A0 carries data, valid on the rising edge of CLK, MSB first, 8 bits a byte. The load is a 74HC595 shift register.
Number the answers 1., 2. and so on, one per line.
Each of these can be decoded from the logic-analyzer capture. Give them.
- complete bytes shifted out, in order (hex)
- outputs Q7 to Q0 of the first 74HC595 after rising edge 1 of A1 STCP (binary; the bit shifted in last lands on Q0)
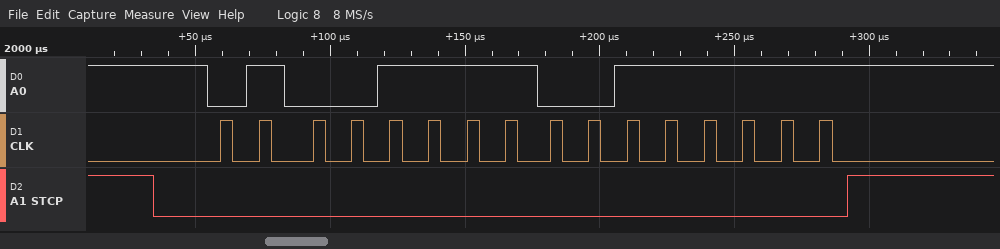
1. 4F 3F
2. 00111111
